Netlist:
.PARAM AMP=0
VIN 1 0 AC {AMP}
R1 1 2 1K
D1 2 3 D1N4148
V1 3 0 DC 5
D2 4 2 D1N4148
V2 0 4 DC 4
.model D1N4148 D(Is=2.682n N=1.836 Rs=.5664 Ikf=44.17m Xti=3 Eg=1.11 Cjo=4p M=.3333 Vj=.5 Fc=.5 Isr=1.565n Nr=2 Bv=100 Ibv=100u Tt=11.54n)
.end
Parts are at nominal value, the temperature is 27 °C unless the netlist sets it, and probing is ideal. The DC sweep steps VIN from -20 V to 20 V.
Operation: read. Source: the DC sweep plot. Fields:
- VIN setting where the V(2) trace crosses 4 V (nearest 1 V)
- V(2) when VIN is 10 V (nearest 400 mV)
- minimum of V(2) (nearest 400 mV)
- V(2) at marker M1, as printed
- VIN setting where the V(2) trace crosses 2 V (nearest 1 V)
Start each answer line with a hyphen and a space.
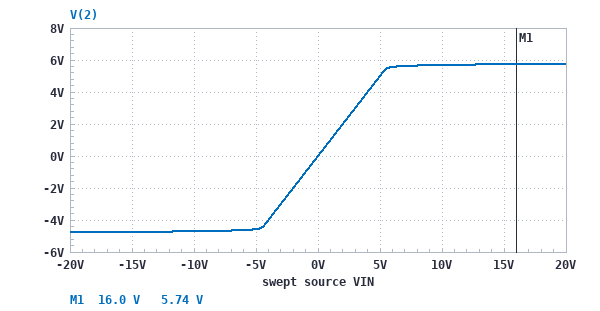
- 4 V
- 5.6 V
- -4.8 V
- 5.74 V
- 2 V
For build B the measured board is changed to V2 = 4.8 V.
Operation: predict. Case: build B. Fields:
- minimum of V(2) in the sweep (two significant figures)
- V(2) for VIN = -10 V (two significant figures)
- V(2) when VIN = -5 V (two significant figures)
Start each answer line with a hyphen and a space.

- -5.6 V
- -5.5 V
- -5.0 V
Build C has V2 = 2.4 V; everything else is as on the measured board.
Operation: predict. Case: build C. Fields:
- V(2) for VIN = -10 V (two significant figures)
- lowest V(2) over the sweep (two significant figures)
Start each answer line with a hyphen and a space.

- -3.1 V
- -3.2 V
